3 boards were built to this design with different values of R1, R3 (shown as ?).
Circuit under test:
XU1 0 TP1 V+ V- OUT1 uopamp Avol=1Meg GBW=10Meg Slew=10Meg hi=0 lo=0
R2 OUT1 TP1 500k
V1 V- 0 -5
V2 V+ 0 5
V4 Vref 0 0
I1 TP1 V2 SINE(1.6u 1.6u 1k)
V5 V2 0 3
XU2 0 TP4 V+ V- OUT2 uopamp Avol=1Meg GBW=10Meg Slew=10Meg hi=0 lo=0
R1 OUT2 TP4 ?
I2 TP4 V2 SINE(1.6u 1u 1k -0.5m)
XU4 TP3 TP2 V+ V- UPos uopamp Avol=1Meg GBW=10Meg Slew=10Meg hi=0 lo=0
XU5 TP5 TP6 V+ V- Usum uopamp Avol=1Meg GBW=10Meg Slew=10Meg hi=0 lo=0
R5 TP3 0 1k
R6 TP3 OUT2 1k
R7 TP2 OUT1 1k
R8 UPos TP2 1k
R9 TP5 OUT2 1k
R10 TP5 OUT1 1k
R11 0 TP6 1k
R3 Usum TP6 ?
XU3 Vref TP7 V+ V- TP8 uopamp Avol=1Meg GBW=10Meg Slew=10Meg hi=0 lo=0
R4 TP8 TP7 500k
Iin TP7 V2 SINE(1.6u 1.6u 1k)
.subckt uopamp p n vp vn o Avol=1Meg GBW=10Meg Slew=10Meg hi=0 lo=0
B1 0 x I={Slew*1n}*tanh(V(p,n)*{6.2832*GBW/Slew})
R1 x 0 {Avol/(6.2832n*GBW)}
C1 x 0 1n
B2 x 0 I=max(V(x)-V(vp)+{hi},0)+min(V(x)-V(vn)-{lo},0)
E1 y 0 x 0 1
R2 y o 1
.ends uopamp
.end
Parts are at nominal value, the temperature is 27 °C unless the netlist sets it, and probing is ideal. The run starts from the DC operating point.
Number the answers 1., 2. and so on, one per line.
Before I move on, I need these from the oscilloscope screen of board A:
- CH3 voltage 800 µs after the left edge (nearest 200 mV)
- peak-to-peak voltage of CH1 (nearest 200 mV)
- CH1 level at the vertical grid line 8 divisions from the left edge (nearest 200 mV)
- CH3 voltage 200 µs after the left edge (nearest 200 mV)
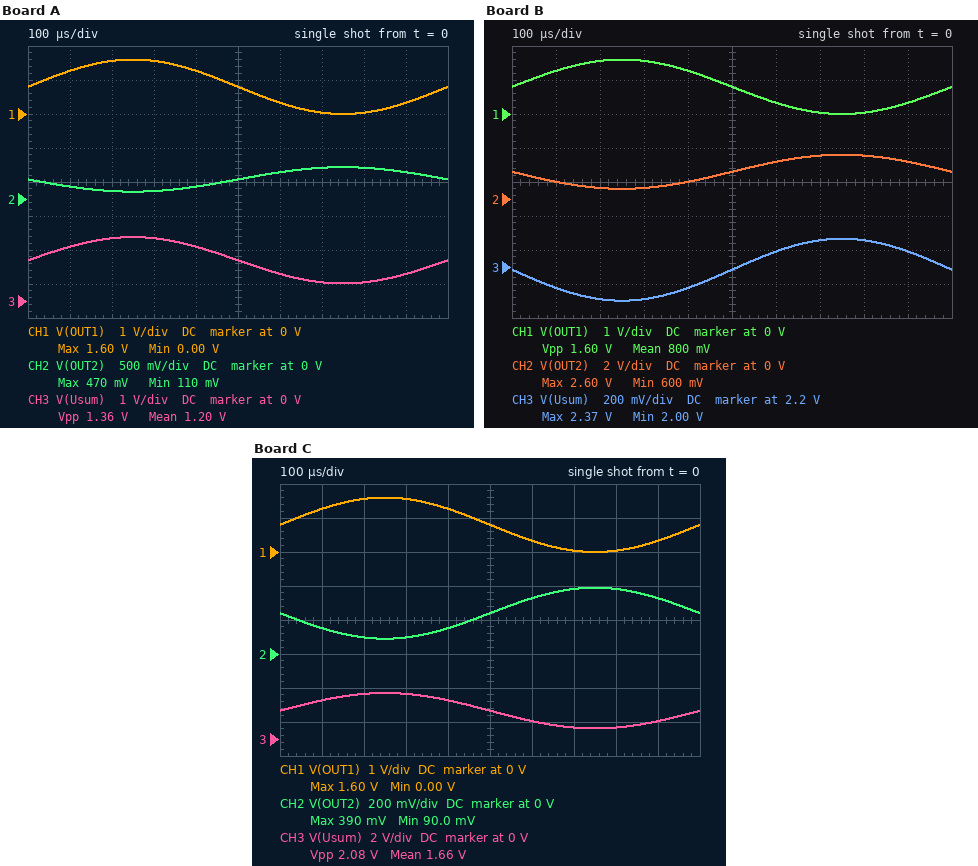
1. 600 mV
2. 1.6 V
3. 0 V
4. 1.8 V
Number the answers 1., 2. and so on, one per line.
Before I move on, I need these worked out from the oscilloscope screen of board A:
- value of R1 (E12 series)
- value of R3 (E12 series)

1. 180 kΩ
2. 1.2 kΩ
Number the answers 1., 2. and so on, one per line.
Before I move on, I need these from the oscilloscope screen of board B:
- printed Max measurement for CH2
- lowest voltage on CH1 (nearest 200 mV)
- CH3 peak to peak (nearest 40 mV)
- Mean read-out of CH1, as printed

1. 2.60 V
2. 0 V
3. 360 mV
4. 800 mV
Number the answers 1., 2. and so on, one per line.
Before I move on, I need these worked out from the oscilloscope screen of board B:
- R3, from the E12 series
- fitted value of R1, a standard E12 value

1. 820 Ω
2. 1 MΩ
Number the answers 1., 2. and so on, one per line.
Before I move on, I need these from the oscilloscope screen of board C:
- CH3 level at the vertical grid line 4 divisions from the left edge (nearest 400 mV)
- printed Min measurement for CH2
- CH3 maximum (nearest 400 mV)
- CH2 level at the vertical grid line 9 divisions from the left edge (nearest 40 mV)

1. 2.4 V
2. 90.0 mV
3. 2.8 V
4. 320 mV
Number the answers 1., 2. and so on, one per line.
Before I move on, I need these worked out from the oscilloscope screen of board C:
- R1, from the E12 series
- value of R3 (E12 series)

1. 150 kΩ
2. 2.2 kΩ
